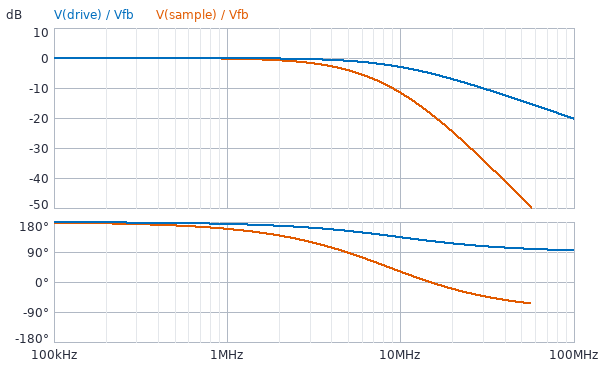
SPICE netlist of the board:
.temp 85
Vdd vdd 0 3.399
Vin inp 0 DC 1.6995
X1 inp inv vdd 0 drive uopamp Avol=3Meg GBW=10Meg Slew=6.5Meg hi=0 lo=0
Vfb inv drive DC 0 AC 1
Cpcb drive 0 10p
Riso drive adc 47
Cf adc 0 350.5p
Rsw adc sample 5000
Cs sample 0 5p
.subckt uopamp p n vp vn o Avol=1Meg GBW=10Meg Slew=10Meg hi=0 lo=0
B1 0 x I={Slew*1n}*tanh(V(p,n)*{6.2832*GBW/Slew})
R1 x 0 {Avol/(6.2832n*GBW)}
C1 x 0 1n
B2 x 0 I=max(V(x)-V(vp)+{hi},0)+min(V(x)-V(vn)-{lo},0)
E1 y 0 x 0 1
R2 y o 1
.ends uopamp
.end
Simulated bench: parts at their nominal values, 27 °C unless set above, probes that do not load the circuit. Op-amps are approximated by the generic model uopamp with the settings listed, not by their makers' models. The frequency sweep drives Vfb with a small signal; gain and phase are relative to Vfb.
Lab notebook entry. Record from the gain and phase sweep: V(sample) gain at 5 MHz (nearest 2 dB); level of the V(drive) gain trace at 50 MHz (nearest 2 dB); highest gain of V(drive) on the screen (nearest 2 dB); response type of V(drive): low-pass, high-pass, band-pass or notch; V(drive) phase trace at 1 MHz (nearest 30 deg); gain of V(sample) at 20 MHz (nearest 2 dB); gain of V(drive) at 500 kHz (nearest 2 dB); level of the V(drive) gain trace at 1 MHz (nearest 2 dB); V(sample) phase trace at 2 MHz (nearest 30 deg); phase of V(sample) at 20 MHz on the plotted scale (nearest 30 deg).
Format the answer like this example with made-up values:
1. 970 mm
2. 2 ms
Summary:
1. -4 dB
2. -14 dB
3. 0 dB
4. low-pass
5. 180 deg
6. -24 dB
7. 0 dB
8. 0 dB
9. 150 deg
10. -30 deg
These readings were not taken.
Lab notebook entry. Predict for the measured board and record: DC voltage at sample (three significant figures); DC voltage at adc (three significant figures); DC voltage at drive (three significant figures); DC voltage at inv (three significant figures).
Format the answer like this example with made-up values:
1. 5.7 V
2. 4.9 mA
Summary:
1. 1.70 V
2. 1.70 V
3. 1.70 V
4. 1.70 V
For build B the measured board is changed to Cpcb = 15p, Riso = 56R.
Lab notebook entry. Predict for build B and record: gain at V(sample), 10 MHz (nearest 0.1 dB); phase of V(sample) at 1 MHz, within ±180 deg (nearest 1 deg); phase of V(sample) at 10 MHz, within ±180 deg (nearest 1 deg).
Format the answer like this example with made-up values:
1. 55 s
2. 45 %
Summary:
1. -12.5 dB
2. 158 deg
3. 26 deg
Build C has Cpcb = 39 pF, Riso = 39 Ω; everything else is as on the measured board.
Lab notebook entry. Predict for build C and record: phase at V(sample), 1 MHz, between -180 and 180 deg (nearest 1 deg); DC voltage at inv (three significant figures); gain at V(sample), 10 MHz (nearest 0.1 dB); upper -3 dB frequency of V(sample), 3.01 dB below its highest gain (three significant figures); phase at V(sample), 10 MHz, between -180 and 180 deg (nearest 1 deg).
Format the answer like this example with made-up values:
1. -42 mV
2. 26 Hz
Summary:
1. 160 deg
2. 1.70 V
3. -10.8 dB
4. 4.37 MHz
5. 36 deg
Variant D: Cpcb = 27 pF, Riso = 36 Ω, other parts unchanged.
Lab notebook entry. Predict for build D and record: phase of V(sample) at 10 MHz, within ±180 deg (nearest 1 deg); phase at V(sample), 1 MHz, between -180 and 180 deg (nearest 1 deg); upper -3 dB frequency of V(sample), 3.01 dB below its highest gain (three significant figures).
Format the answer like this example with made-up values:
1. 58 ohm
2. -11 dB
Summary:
1. 38 deg
2. 161 deg
3. 4.44 MHz
